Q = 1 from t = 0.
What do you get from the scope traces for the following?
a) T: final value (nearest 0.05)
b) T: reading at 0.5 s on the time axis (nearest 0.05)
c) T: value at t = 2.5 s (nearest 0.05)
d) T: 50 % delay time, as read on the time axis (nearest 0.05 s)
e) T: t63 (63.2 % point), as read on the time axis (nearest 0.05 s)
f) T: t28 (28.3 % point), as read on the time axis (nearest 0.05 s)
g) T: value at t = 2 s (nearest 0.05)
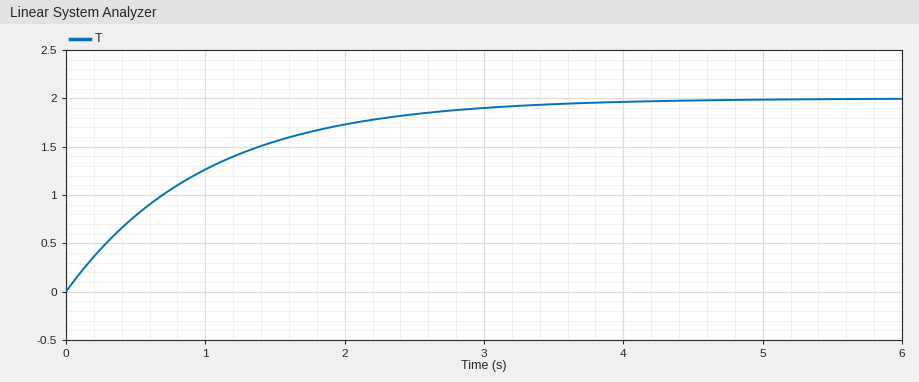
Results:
2.00
0.80
1.85
0.70 s
1.00 s
0.35 s
1.75
